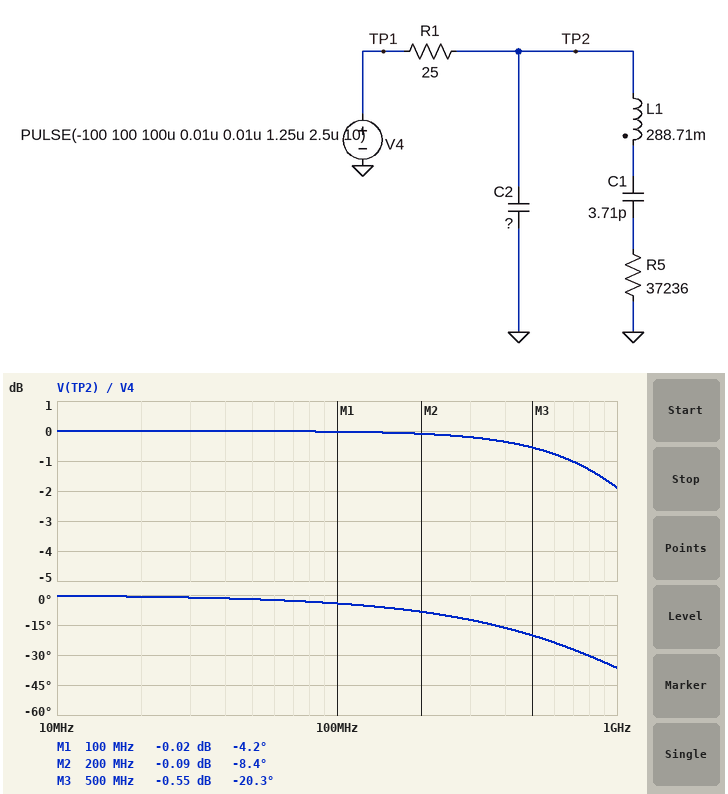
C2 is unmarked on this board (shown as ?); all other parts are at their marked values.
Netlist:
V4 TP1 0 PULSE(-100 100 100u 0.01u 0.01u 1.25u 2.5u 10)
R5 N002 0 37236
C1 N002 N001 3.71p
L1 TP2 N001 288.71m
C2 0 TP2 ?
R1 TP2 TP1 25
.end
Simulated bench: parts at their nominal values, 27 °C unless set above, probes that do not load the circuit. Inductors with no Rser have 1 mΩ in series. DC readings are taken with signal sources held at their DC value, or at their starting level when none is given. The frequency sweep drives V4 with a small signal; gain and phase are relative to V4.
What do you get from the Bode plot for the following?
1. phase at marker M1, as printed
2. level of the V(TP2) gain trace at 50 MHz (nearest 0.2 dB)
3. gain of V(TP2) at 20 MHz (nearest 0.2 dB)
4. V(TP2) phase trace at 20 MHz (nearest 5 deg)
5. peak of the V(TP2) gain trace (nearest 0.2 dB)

-4.2 deg
0 dB
0 dB
0 deg
0 dB
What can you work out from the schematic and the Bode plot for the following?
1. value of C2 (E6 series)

4.7 pF
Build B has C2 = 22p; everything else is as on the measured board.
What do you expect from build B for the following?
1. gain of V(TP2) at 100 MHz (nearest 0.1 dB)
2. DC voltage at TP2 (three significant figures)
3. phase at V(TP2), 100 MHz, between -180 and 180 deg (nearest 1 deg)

-0.5 dB
-100 V
-19 deg
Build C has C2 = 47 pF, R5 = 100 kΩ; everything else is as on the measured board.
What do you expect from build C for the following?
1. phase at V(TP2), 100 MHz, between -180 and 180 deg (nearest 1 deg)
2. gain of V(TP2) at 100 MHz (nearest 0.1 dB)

-36 deg
-1.9 dB
